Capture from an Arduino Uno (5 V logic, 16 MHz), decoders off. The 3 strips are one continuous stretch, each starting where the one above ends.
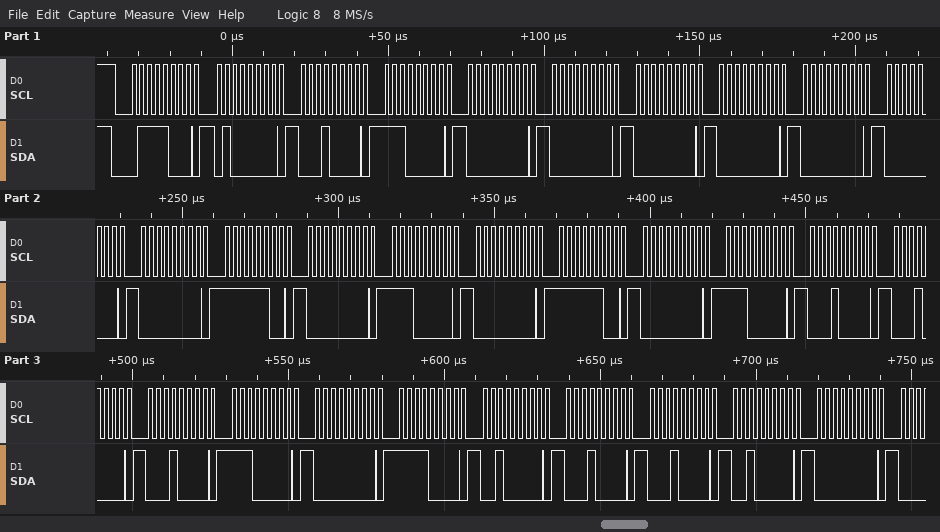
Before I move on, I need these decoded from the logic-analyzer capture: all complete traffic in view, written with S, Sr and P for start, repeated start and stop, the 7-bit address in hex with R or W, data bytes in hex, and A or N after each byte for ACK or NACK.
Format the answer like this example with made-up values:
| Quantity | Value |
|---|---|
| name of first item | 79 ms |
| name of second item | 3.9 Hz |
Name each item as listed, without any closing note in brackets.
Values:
| Quantity | Value |
|---|---|
| all complete traffic in view, written with S, Sr and P for start, repeated start and stop, the 7-bit address in hex with R or W, data bytes in hex, and A or N after each byte for ACK or NACK | S 3CW A 40 A 10 A E0 A 00 A 00 A 00 A 00 A 00 A 00 A 00 A FC A 00 A E0 A 00 A FC A 00 A E0 A 10 A 10 A 10 A E0 A 00 A F0 A 20 A 10 A 10 A 20 A 00 A |
